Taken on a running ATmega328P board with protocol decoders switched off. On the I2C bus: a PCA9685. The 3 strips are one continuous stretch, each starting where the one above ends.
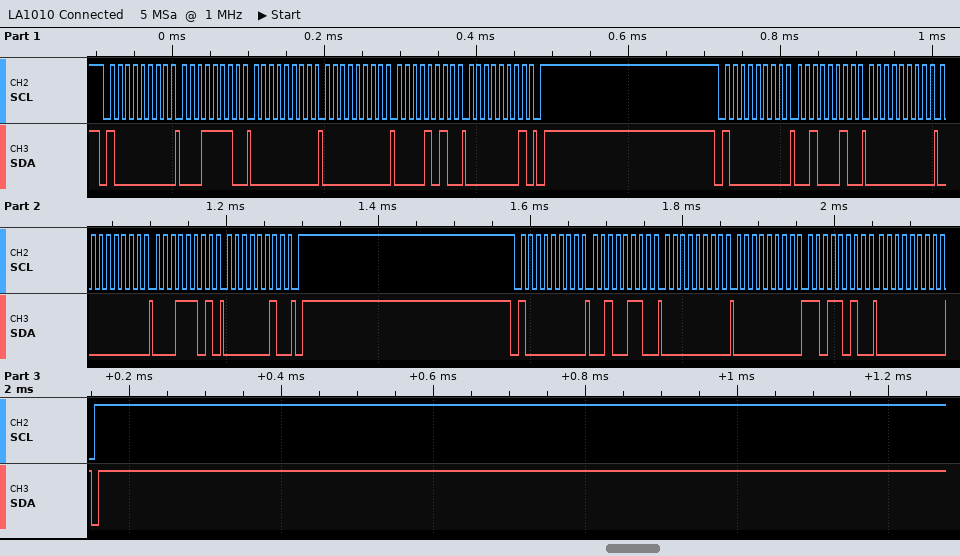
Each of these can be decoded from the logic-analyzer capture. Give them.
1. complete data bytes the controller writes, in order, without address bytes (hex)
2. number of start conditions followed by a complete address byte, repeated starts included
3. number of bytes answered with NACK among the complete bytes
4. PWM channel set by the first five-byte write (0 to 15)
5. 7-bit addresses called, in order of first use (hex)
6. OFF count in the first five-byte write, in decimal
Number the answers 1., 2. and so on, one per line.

1. 1E 00 00 0A 01 22 00 00 1D 02 26 00 00 DA 00
2. 3
3. 0
4. 6
5. 0x40
6. 266
